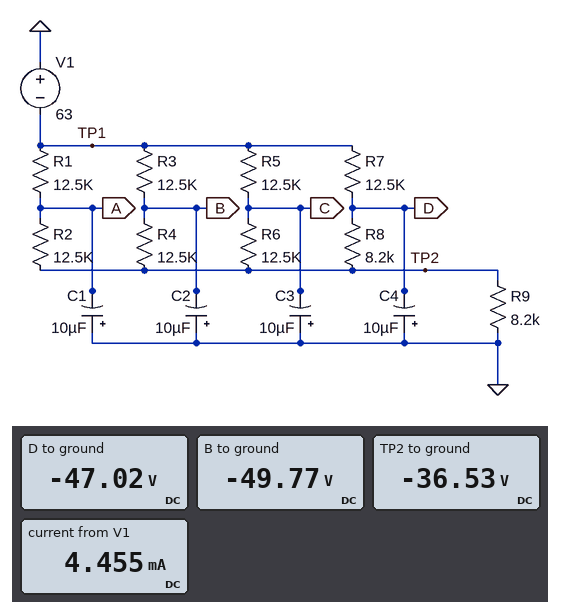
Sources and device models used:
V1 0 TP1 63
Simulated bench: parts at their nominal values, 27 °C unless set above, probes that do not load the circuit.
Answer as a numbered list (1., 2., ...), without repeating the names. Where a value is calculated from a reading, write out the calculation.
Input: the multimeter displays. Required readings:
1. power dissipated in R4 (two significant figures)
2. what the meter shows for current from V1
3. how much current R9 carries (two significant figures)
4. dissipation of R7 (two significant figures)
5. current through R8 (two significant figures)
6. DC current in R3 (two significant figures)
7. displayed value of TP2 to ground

1. (-36.53 V - (-49.77 V))^2 / 12.5 kΩ = 14 mW
2. 4.455 mA
3. (0 V - (-36.53 V)) / 8.2 kΩ = 4.5 mA
4. (-47.02 V - (-63 V))^2 / 12.5 kΩ = 20 mW
5. (-36.53 V - (-47.02 V)) / 8.2 kΩ = 1.3 mA
6. (-49.77 V - (-63 V)) / 12.5 kΩ = 1.1 mA
7. -36.53 V
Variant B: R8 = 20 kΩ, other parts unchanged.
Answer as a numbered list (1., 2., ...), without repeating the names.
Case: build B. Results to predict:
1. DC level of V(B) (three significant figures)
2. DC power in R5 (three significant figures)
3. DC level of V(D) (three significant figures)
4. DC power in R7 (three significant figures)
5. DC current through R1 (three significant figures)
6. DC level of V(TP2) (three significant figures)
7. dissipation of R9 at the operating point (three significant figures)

1. -48.9 V
2. 15.9 mW
3. -52.2 V
4. 9.39 mW
5. 1.13 mA
6. -34.8 V
7. 148 mW
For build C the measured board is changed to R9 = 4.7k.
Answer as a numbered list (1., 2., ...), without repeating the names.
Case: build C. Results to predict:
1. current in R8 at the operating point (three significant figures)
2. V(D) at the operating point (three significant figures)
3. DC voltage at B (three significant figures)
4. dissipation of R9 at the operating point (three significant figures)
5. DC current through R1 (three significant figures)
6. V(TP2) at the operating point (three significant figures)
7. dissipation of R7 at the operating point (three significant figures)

1. 1.70 mA
2. -41.8 V
3. -45.4 V
4. 165 mW
5. 1.41 mA
6. -27.8 V
7. 36.1 mW
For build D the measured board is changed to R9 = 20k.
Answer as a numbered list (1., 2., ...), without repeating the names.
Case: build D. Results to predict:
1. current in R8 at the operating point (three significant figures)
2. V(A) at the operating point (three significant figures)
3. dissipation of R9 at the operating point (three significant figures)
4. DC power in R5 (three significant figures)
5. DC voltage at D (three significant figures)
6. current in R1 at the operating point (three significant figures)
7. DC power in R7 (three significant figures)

1. 697 µA
2. -55.8 V
3. 118 mW
4. 4.16 mW
5. -54.3 V
6. 577 µA
7. 6.07 mW
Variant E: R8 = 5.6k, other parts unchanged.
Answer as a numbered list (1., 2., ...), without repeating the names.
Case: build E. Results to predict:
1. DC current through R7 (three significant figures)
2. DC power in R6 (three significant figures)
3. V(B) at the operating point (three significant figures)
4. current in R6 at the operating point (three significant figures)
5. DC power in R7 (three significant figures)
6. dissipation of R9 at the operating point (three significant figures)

1. 1.43 mA
2. 13.4 mW
3. -50.1 V
4. 1.03 mA
5. 25.5 mW
6. 168 mW
